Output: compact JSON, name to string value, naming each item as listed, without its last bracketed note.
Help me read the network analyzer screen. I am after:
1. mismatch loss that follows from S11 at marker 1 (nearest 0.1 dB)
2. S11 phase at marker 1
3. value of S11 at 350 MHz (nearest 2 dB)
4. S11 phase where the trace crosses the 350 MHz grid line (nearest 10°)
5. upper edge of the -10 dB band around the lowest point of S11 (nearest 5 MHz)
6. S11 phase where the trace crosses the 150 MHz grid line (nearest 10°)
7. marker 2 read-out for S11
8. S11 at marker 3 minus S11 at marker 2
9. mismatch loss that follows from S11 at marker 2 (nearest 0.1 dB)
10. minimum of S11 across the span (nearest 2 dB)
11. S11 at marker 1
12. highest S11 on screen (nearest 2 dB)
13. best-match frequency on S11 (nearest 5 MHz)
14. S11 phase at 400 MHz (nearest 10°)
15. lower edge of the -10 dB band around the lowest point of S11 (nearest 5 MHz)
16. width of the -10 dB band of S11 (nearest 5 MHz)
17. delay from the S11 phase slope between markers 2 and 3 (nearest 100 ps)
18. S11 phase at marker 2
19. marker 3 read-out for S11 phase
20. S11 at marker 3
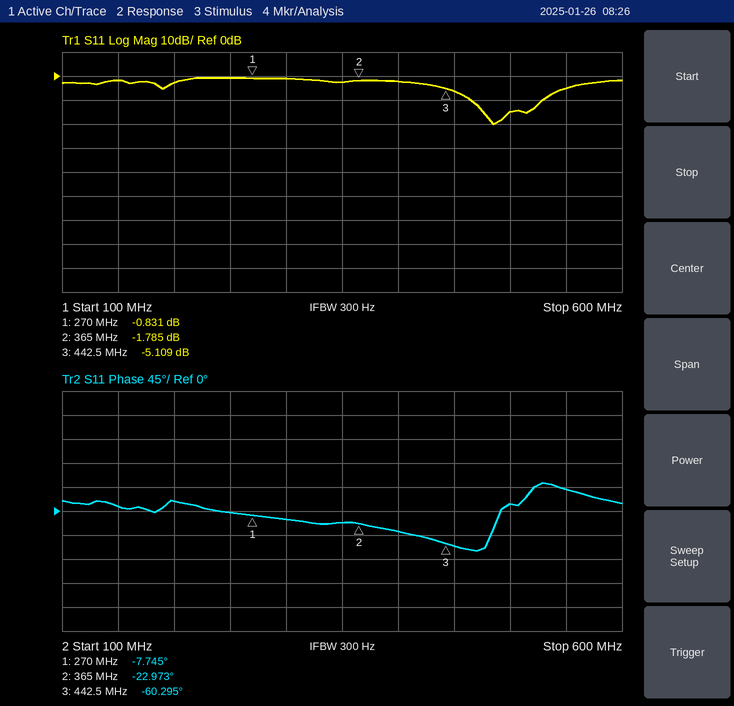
{"mismatch loss that follows from S11 at marker 1": "7.6 dB", "S11 phase at marker 1": "-7.745°", "value of S11 at 350 MHz": "-2 dB", "S11 phase where the trace crosses the 350 MHz grid line": "-20°", "upper edge of the -10 dB band around the lowest point of S11": "530 MHz", "S11 phase where the trace crosses the 150 MHz grid line": "10°", "marker 2 read-out for S11": "-1.785 dB", "S11 at marker 3 minus S11 at marker 2": "-3.324 dB", "mismatch loss that follows from S11 at marker 2": "4.7 dB", "minimum of S11 across the span": "-20 dB", "S11 at marker 1": "-0.831 dB", "highest S11 on screen": "0 dB", "best-match frequency on S11": "485 MHz", "S11 phase at 400 MHz": "-40°", "lower edge of the -10 dB band around the lowest point of S11": "465 MHz", "width of the -10 dB band of S11": "65 MHz", "delay from the S11 phase slope between markers 2 and 3": "1.3 ns", "S11 phase at marker 2": "-22.973°", "marker 3 read-out for S11 phase": "-60.295°", "S11 at marker 3": "-5.109 dB"}
